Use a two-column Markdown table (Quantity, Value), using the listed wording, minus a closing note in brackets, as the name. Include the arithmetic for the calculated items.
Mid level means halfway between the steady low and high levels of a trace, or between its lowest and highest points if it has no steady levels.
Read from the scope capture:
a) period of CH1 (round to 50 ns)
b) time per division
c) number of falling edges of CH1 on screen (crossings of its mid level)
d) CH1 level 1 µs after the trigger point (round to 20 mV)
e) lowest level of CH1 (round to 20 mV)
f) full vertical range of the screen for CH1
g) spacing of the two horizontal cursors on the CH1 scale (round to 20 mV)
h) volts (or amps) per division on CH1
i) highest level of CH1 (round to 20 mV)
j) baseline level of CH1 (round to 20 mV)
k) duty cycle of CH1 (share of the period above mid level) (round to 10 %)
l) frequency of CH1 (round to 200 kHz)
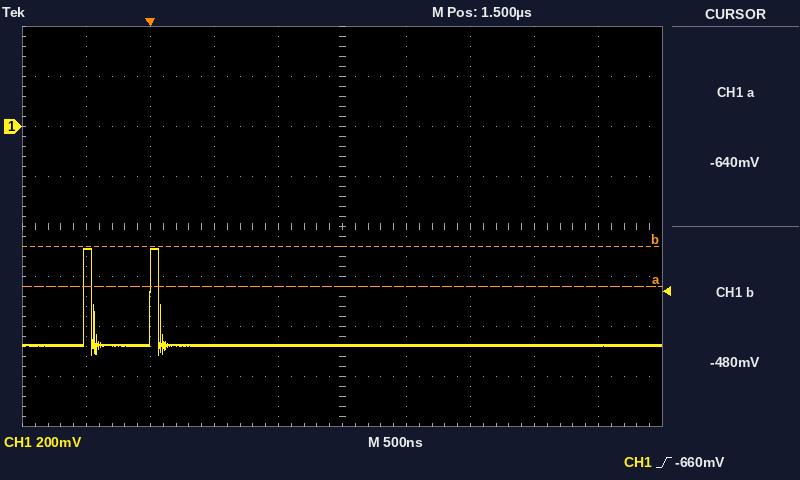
| Quantity | Value |
|---|---|
| period of CH1 | 500 ns |
| time per division | 500 ns |
| number of falling edges of CH1 on screen | 2 |
| CH1 level 1 µs after the trigger point | -880 mV |
| lowest level of CH1 | -920 mV |
| full vertical range of the screen for CH1 | 1.6 V |
| spacing of the two horizontal cursors on the CH1 scale | 160 mV |
| volts (or amps) per division on CH1 | 200 mV |
| highest level of CH1 | -480 mV |
| baseline level of CH1 | -880 mV |
| duty cycle of CH1 (share of the period above mid level) | 10 % |
| frequency of CH1 | 1 / 500 ns ≈ 2.0 MHz |
